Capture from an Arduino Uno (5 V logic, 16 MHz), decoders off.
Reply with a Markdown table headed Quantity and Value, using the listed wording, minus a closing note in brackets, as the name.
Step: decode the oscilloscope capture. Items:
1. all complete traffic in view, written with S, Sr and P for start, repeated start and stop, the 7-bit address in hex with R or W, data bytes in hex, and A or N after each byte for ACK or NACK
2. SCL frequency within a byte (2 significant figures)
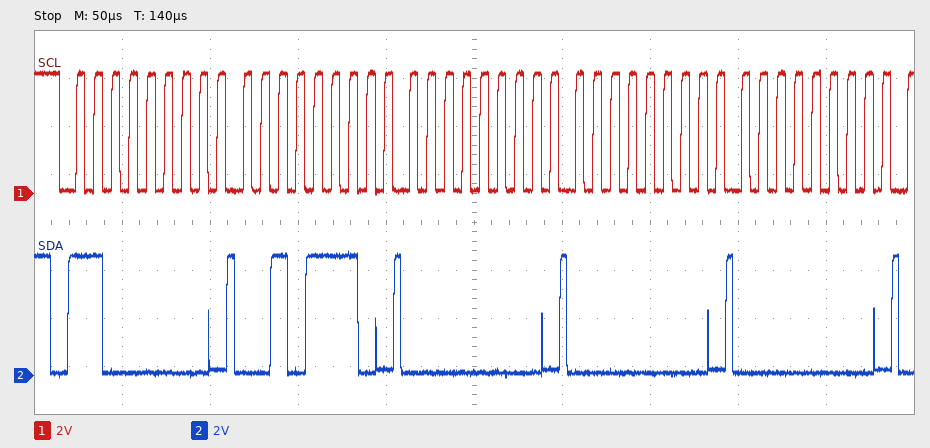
| Quantity | Value |
|---|---|
| all complete traffic in view, written with S, Sr and P for start, repeated start and stop, the 7-bit address in hex with R or W, data bytes in hex, and A or N after each byte for ACK or NACK | S 60W A 2E A 00 A 00 A 00 A |
| SCL frequency within a byte | 100 kHz |
